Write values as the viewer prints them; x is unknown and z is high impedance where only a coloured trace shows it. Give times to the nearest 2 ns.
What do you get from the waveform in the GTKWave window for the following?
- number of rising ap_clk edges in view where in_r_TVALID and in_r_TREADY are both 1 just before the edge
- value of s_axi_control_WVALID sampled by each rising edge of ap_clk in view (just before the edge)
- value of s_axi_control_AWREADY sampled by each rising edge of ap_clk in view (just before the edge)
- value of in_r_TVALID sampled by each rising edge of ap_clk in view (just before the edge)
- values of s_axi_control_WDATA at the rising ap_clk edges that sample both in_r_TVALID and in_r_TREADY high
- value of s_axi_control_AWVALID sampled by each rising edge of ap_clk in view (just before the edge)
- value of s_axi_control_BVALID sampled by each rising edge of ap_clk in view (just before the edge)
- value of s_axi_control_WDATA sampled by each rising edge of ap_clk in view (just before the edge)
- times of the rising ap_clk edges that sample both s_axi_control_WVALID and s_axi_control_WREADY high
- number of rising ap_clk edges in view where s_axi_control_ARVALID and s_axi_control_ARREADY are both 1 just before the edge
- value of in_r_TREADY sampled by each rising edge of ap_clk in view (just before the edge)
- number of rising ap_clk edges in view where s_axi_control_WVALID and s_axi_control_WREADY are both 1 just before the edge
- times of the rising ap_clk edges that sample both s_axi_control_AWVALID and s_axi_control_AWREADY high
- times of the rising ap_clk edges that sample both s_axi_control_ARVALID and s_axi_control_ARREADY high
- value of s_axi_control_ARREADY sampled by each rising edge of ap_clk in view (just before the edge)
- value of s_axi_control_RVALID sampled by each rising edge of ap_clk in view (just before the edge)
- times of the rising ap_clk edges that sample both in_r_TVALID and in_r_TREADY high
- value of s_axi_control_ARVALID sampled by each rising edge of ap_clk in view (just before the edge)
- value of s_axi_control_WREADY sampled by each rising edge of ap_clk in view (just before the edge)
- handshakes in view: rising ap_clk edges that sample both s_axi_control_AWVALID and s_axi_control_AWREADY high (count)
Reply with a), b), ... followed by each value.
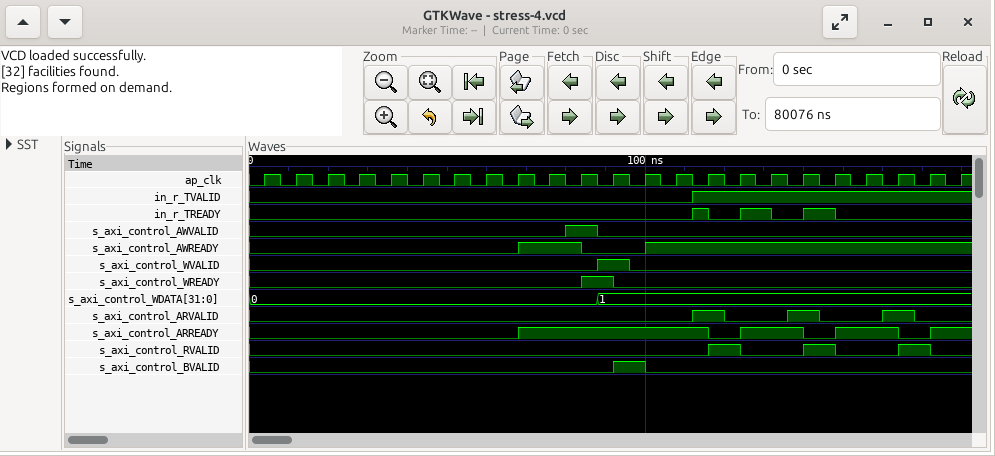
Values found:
a) 3
b) 0 0 0 0 0 0 0 0 0 0 0 1 0 0 0 0 0 0 0 0 0 0 0
c) 0 0 0 0 0 0 0 0 0 1 1 0 0 1 1 1 1 1 1 1 1 1 1
d) 0 0 0 0 0 0 0 0 0 0 0 0 0 0 1 1 1 1 1 1 1 1 1
e) 1, 1, 1
f) 0 0 0 0 0 0 0 0 0 0 1 0 0 0 0 0 0 0 0 0 0 0 0
g) 0 0 0 0 0 0 0 0 0 0 0 0 1 0 0 0 0 0 0 0 0 0 0
h) 0, 0, 0, 0, 0, 0, 0, 0, 0, 0, 0, 1, 1, 1, 1, 1, 1, 1, 1, 1, 1, 1, 1
i) 92 ns
j) 3
k) 0 0 0 0 0 0 0 0 0 0 0 0 0 0 1 0 1 0 1 0 0 0 0
l) 1
m) 84 ns
n) 116 ns, 140 ns, 164 ns
o) 0 0 0 0 0 0 0 0 0 1 1 1 1 1 1 0 1 1 0 1 1 0 1
p) 0 0 0 0 0 0 0 0 0 0 0 0 0 0 0 1 0 0 1 0 0 1 0
q) 116 ns, 132 ns, 148 ns
r) 0 0 0 0 0 0 0 0 0 0 0 0 0 0 1 0 0 1 0 0 1 0 0
s) 0 0 0 0 0 0 0 0 0 0 0 1 0 0 0 0 0 0 0 0 0 0 0
t) 1
